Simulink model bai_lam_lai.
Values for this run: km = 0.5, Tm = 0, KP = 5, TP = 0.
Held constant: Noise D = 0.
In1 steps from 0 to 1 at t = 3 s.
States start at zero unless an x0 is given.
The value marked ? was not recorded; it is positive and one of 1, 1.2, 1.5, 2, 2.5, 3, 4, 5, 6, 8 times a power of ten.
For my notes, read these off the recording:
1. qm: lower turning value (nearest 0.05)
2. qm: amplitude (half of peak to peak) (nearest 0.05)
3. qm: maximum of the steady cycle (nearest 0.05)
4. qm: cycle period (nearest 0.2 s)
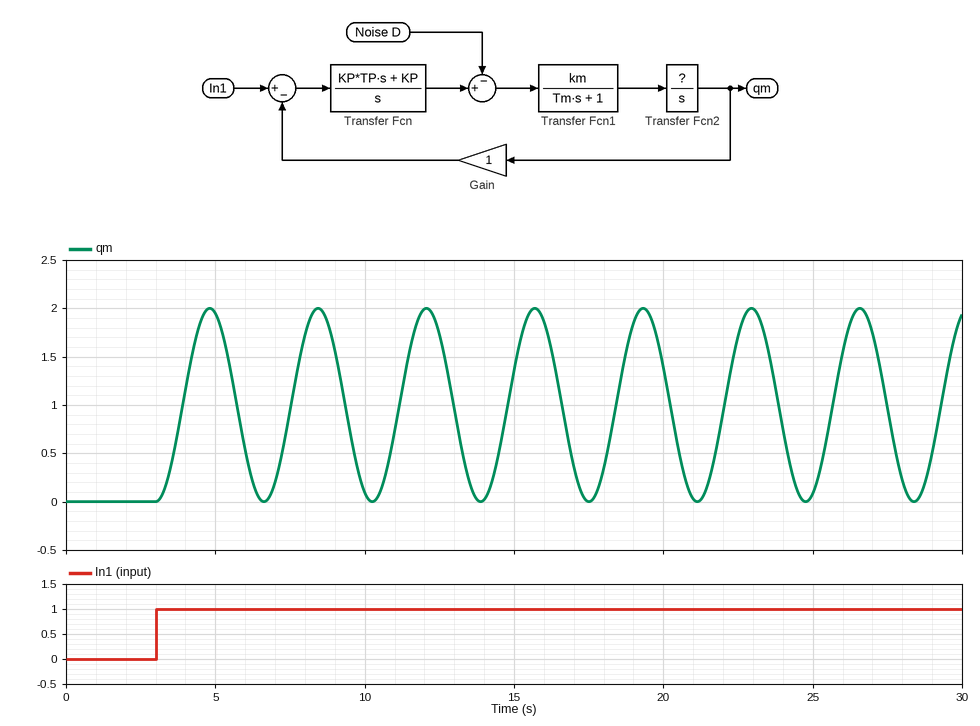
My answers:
0.00
1.00
2.00
3.6 s
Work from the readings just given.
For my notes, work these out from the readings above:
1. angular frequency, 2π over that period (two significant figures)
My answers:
1.7 rad/s
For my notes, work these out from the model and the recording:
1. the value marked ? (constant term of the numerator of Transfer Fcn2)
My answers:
1.2
